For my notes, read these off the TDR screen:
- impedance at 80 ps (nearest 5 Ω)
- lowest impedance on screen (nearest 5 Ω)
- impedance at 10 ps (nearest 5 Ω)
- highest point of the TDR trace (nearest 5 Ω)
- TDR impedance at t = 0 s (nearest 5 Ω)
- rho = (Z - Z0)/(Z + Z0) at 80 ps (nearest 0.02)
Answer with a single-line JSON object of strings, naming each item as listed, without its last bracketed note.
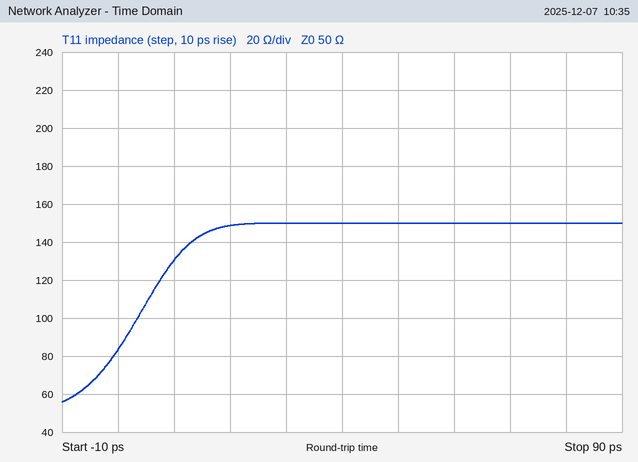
{"impedance at 80 ps": "150 Ω", "lowest impedance on screen": "55 Ω", "impedance at 10 ps": "130 Ω", "highest point of the TDR trace": "150 Ω", "TDR impedance at t = 0 s": "85 Ω", "rho = (Z - Z0)/(Z + Z0) at 80 ps": "+0.50"}
